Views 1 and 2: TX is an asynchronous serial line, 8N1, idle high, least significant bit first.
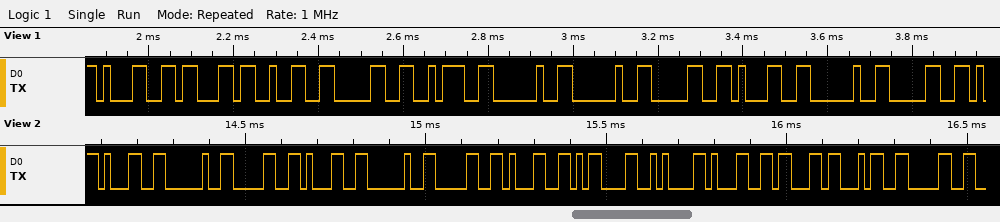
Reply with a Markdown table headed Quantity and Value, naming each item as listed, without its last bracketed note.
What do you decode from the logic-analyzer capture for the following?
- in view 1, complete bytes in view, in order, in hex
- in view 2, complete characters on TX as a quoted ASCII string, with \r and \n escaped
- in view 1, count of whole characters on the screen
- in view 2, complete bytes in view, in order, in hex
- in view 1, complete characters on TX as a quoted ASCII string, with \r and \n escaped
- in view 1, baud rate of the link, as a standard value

| Quantity | Value |
|---|---|
| in view 1, complete bytes in view, in order, in hex | 0x31 0x63 0x32 0x30 0x3A 0x20 0x20 0x30 0x31 0x20 0x30 |
| in view 2, complete characters on TX as a quoted ASCII string, with \r and \n escaped | "1 01 01\r\n1c40" |
| in view 1, count of whole characters on the screen | 11 |
| in view 2, complete bytes in view, in order, in hex | 31 20 30 31 20 30 31 0D 0A 31 63 34 30 |
| in view 1, complete characters on TX as a quoted ASCII string, with \r and \n escaped | "1c20:  01 0" |
| in view 1, baud rate of the link, as a standard value | 57600 baud |
